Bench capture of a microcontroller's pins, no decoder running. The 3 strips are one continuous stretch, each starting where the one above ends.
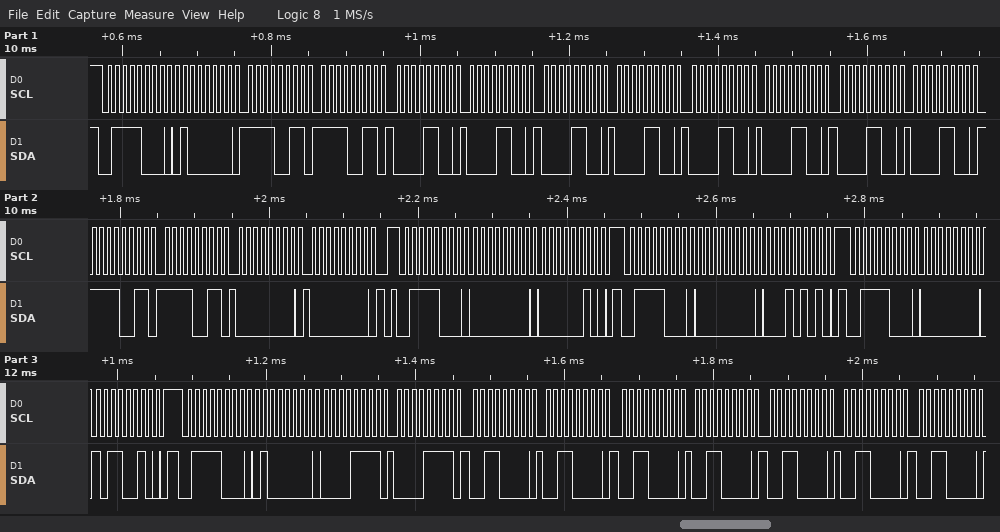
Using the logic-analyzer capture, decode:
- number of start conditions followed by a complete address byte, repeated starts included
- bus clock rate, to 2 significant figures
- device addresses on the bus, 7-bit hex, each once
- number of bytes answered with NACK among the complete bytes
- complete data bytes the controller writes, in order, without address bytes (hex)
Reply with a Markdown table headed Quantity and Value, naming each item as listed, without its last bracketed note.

| Quantity | Value |
|---|---|
| number of start conditions followed by a complete address byte, repeated starts included | 5 |
| bus clock rate, to 2 significant figures | 100 kHz |
| device addresses on the bus, 7-bit hex, each once | 0x3C |
| number of bytes answered with NACK among the complete bytes | 0 |
| complete data bytes the controller writes, in order, without address bytes | 40 F3 F3 0C 0C 0C 0C 0C 0C 0C 0C F3 F3 00 00 00 02 00 15 00 B2 40 0F 0F 30 30 30 30 30 30 30 |
